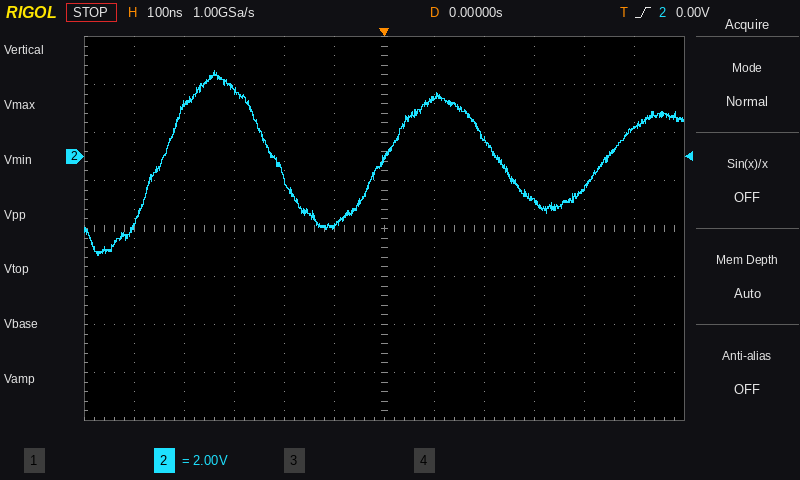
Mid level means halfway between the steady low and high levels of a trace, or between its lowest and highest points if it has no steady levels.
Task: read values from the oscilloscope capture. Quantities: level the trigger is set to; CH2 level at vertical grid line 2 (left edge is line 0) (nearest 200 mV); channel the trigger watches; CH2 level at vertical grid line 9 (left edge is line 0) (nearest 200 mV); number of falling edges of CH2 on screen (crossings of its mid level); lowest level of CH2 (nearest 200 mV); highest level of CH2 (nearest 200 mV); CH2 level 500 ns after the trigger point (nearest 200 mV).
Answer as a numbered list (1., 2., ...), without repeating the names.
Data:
1. 0.00 V
2. 2.2 V
3. CH2
4. -1.8 V
5. 2
6. -4.2 V
7. 3.6 V
8. 1.2 V
